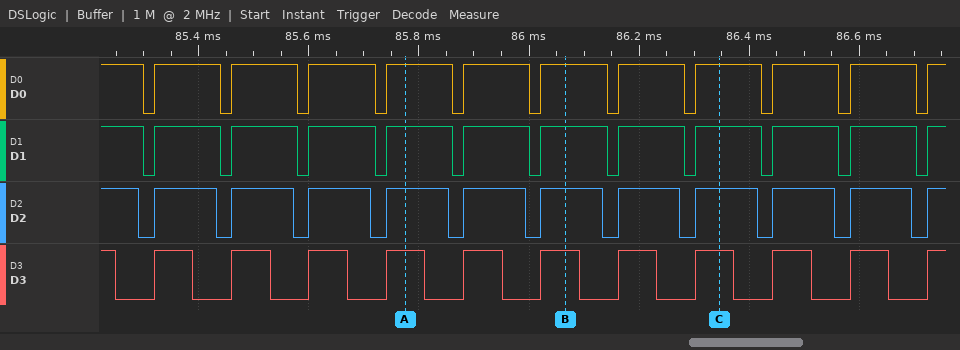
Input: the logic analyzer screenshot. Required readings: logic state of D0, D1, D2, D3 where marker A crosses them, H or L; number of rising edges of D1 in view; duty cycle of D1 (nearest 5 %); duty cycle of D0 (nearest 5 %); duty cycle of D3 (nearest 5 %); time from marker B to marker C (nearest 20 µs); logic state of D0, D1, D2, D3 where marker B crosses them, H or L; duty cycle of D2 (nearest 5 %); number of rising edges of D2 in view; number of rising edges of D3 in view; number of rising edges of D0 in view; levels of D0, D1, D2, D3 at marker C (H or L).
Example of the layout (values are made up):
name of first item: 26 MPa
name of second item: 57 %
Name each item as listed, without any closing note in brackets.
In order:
logic state of D0, D1, D2, D3 where marker A crosses them, H or L: D0=H, D1=H, D2=H, D3=H
number of rising edges of D1 in view: 11
duty cycle of D1: 85 %
duty cycle of D0: 85 %
duty cycle of D3: 50 %
time from marker B to marker C: 280 µs
logic state of D0, D1, D2, D3 where marker B crosses them, H or L: D0=H, D1=H, D2=H, D3=H
duty cycle of D2: 80 %
number of rising edges of D2 in view: 11
number of rising edges of D3 in view: 11
number of rising edges of D0 in view: 11
levels of D0, D1, D2, D3 at marker C: D0=H, D1=H, D2=H, D3=H
